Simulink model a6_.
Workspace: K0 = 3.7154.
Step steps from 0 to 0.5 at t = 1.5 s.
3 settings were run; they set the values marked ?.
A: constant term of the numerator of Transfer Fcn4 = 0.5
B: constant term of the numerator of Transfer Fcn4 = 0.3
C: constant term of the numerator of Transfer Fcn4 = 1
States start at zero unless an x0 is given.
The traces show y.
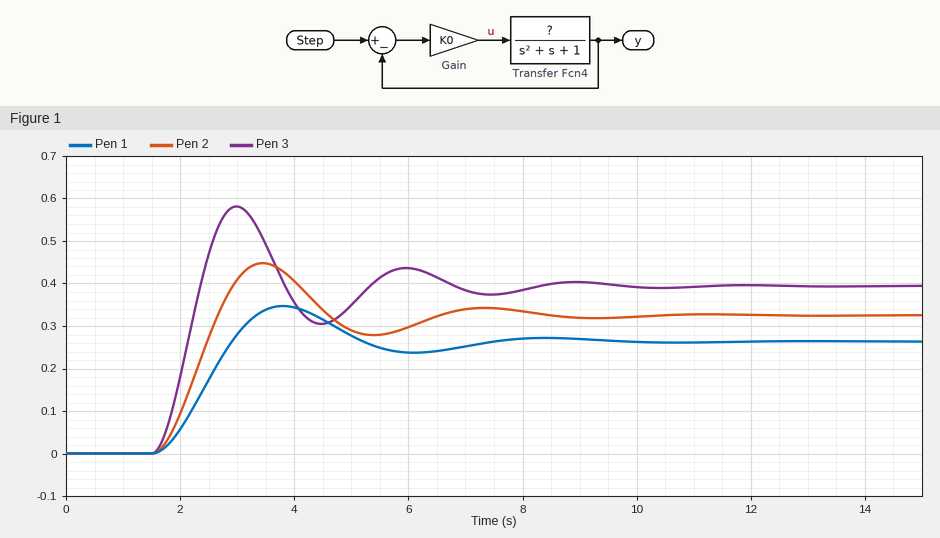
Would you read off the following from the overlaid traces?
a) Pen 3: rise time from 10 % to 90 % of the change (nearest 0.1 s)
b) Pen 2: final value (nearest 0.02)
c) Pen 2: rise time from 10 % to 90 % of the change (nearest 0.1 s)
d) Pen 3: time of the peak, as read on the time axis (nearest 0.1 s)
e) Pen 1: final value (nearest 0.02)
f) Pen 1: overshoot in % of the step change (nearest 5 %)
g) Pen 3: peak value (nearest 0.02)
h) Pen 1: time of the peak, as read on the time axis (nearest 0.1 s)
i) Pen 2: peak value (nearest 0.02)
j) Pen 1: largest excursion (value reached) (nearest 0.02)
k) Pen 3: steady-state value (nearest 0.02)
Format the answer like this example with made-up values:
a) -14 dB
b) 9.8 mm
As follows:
a) 0.6 s
b) 0.32
c) 0.8 s
d) 3.0 s
e) 0.26
f) 30 %
g) 0.58
h) 3.8 s
i) 0.44
j) 0.34
k) 0.40
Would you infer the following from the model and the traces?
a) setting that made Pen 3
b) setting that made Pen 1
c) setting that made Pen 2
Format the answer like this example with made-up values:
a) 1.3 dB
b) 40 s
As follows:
a) C
b) B
c) A
